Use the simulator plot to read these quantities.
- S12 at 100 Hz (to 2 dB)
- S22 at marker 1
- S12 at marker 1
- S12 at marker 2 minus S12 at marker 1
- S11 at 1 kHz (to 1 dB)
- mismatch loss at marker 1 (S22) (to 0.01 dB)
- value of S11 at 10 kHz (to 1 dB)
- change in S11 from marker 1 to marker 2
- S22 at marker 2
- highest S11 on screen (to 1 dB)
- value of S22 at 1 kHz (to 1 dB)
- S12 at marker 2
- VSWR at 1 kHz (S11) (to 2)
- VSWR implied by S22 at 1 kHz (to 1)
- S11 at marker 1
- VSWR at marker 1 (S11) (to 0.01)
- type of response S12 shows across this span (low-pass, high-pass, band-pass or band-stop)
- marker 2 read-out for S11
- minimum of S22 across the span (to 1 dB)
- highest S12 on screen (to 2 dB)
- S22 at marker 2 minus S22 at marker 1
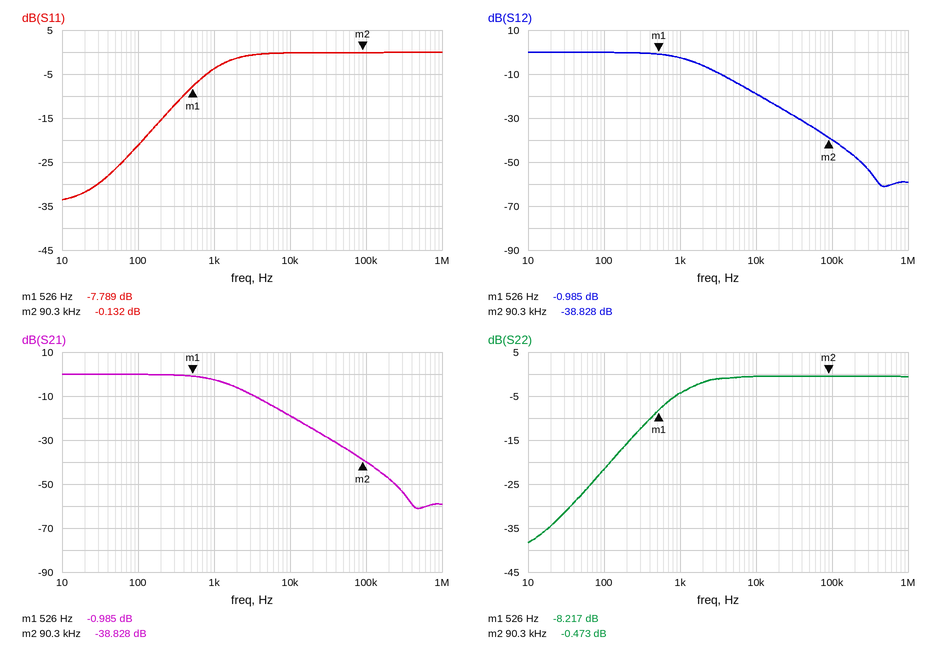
0 dB
-8.217 dB
-0.985 dB
-37.843 dB
-4 dB
0.71 dB
0 dB
7.657 dB
-0.473 dB
0 dB
-4 dB
-38.828 dB
4
4
-7.789 dB
2.38
low-pass
-0.132 dB
-38 dB
0 dB
7.744 dB
